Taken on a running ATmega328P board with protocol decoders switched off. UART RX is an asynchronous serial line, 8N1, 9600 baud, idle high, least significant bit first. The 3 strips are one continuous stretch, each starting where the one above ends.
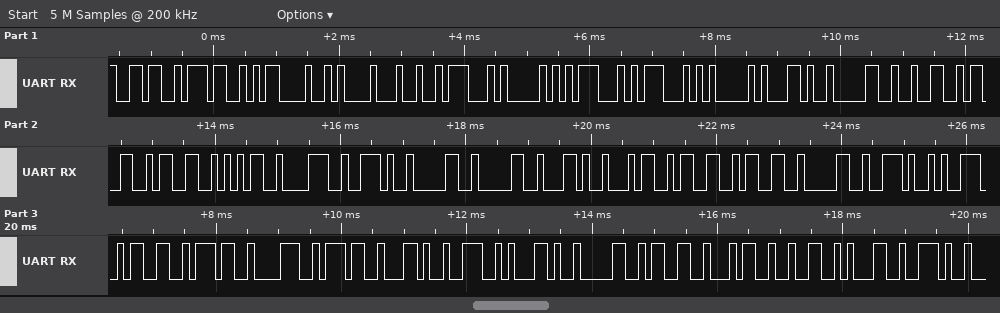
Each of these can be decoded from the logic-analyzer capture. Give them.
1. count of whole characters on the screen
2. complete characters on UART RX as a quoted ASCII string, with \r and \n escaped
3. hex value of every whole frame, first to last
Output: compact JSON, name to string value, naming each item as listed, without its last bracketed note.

{"count of whole characters on the screen": "40", "complete characters on UART RX as a quoted ASCII string, with \\r and \\n escaped": "\"67\\r\\n$GPGGA,023358.00,4330.93787,N,03421.\"", "hex value of every whole frame, first to last": "0x36 0x37 0x0D 0x0A 0x24 0x47 0x50 0x47 0x47 0x41 0x2C 0x30 0x32 0x33 0x33 0x35 0x38 0x2E 0x30 0x30 0x2C 0x34 0x33 0x33 0x30 0x2E 0x39 0x33 0x37 0x38 0x37 0x2C 0x4E 0x2C 0x30 0x33 0x34 0x32 0x31 0x2E"}
